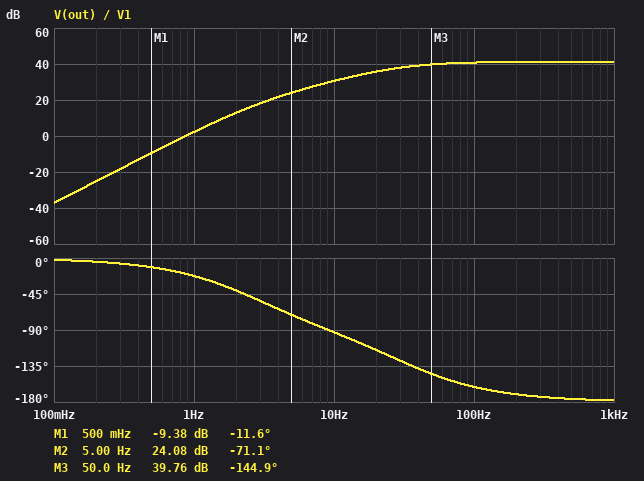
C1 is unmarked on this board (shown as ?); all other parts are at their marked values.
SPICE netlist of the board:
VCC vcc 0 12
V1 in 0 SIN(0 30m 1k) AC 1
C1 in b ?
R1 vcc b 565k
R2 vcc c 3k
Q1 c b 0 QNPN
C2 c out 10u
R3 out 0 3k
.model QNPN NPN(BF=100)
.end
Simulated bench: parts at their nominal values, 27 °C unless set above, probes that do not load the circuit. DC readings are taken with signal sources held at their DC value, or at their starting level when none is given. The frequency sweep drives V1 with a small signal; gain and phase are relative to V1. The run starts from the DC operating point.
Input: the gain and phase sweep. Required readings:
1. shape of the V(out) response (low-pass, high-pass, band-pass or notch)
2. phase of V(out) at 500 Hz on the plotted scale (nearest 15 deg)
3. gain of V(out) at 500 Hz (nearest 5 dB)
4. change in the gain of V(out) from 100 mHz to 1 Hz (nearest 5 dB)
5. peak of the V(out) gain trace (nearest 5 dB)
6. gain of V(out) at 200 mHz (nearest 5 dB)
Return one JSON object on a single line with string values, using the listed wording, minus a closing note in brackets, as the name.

{"shape of the V(out) response": "high-pass", "phase of V(out) at 500 Hz on the plotted scale": "-180 deg", "gain of V(out) at 500 Hz": "40 dB", "change in the gain of V(out) from 100 mHz to 1 Hz": "40 dB", "peak of the V(out) gain trace": "40 dB", "gain of V(out) at 200 mHz": "-25 dB"}
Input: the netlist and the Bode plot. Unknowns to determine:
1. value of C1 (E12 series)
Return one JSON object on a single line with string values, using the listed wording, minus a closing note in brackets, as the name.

{"value of C1": "3.9 µF"}
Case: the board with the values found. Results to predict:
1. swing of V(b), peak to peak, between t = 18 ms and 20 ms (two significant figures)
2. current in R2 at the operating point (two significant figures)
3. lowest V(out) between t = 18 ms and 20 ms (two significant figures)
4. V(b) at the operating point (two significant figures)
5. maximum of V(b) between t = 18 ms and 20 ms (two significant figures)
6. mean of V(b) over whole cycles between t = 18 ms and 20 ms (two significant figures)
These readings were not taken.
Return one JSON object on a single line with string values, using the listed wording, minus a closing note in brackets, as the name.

{"swing of V(b), peak to peak, between t = 18 ms and 20 ms": "60 mV", "current in R2 at the operating point": "2.0 mA", "lowest V(out) between t = 18 ms and 20 ms": "-4.0 V", "V(b) at the operating point": "790 mV", "maximum of V(b) between t = 18 ms and 20 ms": "810 mV", "mean of V(b) over whole cycles between t = 18 ms and 20 ms": "780 mV"}
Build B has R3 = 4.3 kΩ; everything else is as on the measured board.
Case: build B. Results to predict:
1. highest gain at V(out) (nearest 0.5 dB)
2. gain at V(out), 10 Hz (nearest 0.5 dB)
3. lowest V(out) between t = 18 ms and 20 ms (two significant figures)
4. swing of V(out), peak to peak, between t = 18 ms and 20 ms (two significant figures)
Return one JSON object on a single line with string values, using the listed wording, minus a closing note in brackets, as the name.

{"highest gain at V(out)": "42.5 dB", "gain at V(out), 10 Hz": "32.0 dB", "lowest V(out) between t = 18 ms and 20 ms": "-4.7 V", "swing of V(out), peak to peak, between t = 18 ms and 20 ms": "7.4 V"}
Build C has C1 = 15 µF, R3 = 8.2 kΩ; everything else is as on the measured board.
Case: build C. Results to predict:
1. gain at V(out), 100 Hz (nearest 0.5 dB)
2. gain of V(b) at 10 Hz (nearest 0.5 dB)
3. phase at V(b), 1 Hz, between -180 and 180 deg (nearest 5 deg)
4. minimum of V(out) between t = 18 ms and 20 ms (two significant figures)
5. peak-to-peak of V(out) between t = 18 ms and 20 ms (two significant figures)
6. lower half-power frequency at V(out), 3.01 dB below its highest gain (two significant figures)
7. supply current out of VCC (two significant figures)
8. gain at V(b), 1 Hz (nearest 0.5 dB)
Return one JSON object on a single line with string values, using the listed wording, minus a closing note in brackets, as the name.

{"gain at V(out), 100 Hz": "44.5 dB", "gain of V(b) at 10 Hz": "-2.0 dB", "phase at V(b), 1 Hz, between -180 and 180 deg": "85 deg", "minimum of V(out) between t = 18 ms and 20 ms": "-5.8 V", "peak-to-peak of V(out) between t = 18 ms and 20 ms": "9.2 V", "lower half-power frequency at V(out), 3.01 dB below its highest gain": "8.4 Hz", "supply current out of VCC": "2.0 mA", "gain at V(b), 1 Hz": "-18.5 dB"}
